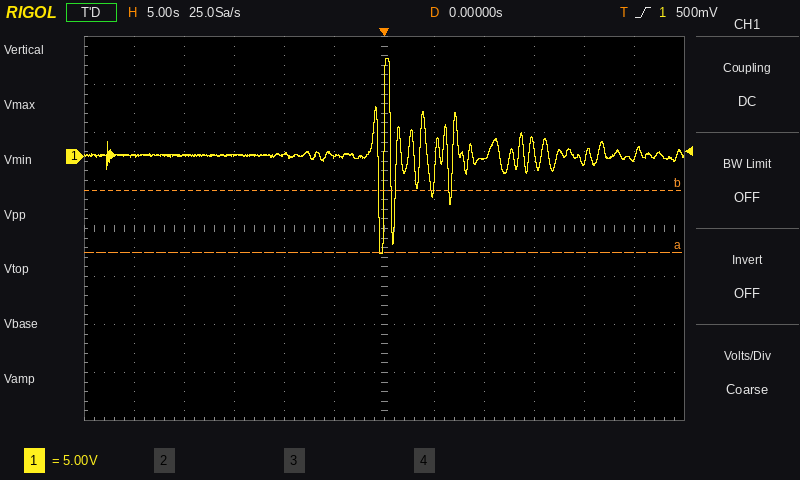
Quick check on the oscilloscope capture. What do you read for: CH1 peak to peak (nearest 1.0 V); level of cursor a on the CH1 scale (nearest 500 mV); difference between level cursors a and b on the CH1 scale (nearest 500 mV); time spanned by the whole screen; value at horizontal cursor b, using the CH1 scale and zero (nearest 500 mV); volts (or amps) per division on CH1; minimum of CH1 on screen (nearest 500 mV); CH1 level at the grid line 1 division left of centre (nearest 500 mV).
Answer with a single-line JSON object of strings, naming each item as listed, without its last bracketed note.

{"CH1 peak to peak": "20.0 V", "level of cursor a on the CH1 scale": "-10.0 V", "difference between level cursors a and b on the CH1 scale": "6.5 V", "time spanned by the whole screen": "60 s", "value at horizontal cursor b, using the CH1 scale and zero": "-3.5 V", "volts (or amps) per division on CH1": "5 V", "minimum of CH1 on screen": "-10.0 V", "CH1 level at the grid line 1 division left of centre": "0.0 V"}
